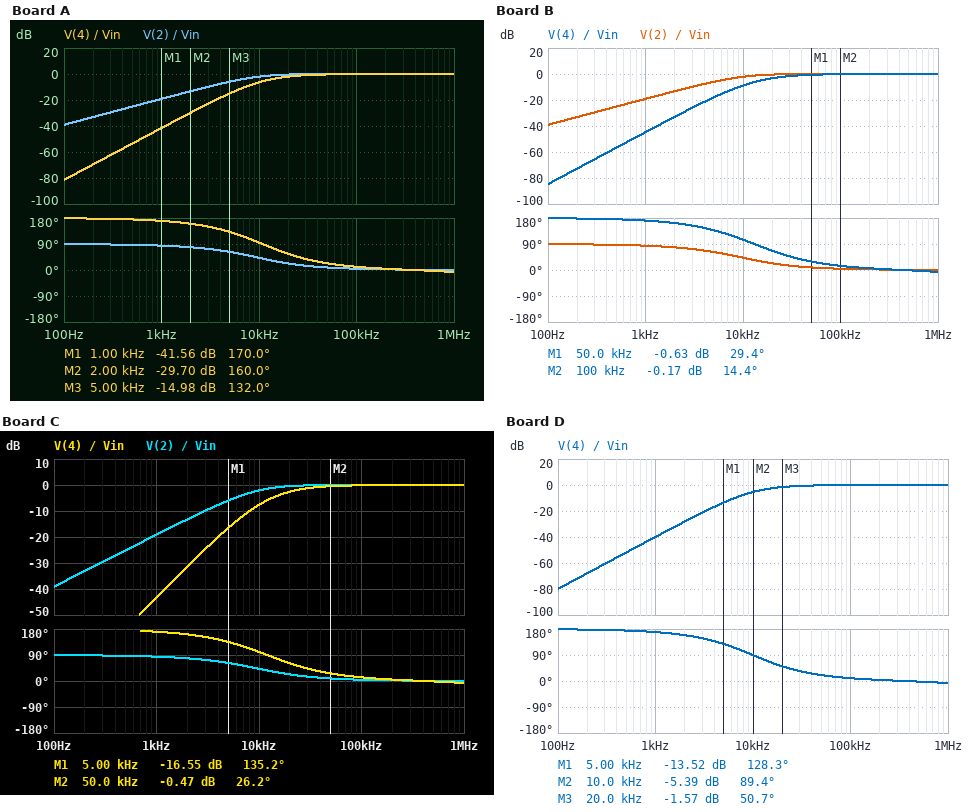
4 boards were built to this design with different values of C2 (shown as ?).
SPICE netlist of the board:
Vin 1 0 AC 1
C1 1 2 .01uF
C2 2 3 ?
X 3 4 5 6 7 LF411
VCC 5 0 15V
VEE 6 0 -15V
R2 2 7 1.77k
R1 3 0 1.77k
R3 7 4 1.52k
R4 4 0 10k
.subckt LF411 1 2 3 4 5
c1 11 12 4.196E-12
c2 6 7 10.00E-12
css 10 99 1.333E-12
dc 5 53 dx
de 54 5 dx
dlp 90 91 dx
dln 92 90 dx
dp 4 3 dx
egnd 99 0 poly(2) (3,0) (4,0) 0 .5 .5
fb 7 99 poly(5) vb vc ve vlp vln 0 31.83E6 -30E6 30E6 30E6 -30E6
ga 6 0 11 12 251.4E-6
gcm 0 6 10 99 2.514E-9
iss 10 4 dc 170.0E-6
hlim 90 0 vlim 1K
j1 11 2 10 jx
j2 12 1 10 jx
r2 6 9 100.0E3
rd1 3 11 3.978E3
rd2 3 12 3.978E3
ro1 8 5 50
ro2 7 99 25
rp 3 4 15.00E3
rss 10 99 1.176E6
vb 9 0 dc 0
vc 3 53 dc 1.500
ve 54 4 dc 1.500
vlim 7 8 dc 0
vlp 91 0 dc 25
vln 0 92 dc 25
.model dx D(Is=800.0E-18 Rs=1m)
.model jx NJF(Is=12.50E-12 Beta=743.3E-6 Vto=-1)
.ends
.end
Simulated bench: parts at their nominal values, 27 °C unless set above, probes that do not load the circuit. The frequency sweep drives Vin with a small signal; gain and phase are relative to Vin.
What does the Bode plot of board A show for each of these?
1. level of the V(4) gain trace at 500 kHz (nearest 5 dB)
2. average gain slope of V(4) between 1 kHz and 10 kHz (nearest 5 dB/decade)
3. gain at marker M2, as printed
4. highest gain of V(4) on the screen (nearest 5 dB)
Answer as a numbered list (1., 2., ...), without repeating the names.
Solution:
1. 0 dB
2. 35 dB/decade
3. -29.70 dB
4. 0 dB
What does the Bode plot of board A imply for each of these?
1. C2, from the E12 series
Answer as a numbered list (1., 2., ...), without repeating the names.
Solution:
1. 6.8 nF
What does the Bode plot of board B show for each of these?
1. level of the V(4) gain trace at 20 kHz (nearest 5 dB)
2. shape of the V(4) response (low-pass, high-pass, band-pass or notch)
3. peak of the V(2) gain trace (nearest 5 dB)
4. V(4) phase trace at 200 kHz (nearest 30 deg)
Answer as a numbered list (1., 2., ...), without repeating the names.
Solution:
1. -5 dB
2. high-pass
3. 0 dB
4. 0 deg
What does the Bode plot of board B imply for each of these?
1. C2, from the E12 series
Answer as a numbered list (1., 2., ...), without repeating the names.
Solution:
1. 4.7 nF
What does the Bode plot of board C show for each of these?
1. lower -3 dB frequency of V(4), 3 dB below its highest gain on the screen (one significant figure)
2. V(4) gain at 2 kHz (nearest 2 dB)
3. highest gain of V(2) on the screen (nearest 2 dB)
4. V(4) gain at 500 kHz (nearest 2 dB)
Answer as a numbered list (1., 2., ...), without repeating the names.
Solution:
1. 20 kHz
2. -32 dB
3. 0 dB
4. 0 dB
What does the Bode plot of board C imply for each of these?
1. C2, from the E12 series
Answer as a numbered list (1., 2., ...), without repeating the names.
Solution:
1. 5.6 nF
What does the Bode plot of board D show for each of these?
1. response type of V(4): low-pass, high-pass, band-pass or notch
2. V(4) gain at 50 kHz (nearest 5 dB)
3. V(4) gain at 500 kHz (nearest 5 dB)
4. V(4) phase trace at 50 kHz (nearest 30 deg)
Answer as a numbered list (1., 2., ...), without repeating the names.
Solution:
1. high-pass
2. 0 dB
3. 0 dB
4. 30 deg
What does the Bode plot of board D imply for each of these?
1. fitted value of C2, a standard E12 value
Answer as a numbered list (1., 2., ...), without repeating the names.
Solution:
1. 8.2 nF
